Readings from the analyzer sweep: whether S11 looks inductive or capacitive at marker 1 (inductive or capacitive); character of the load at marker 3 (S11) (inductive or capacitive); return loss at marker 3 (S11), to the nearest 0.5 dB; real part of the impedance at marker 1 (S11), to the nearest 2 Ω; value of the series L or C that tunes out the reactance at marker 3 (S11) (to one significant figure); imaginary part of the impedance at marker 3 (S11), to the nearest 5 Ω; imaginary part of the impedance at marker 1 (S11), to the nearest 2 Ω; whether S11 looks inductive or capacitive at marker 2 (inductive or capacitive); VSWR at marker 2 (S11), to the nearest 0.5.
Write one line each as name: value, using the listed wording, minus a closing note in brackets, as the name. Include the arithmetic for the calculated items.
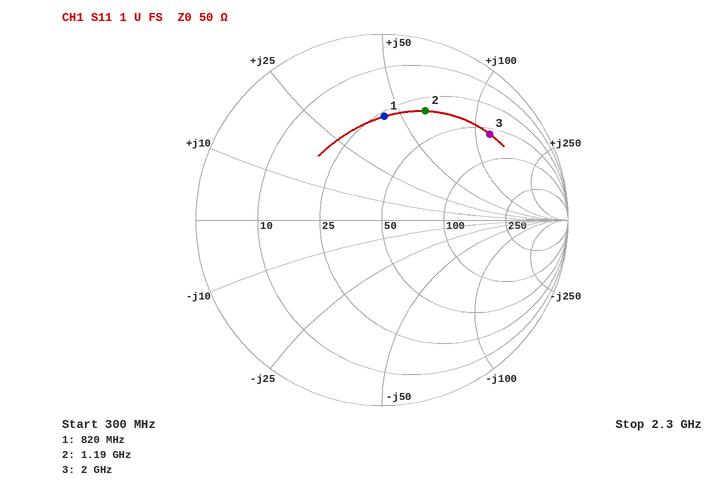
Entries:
whether S11 looks inductive or capacitive at marker 1: inductive
character of the load at marker 3 (S11): inductive
return loss at marker 3 (S11), to the nearest 0.5 dB: 2.5 dB
real part of the impedance at marker 1 (S11), to the nearest 2 Ω: 26 Ω
value of the series L or C that tunes out the reactance at marker 3 (S11): C = 1/(2π × 2 GHz × 120 Ω) ≈ 663 fF, so 700 fF to one significant figure
imaginary part of the impedance at marker 3 (S11), to the nearest 5 Ω: +120 Ω
imaginary part of the impedance at marker 1 (S11), to the nearest 2 Ω: +44 Ω
whether S11 looks inductive or capacitive at marker 2: inductive
VSWR at marker 2 (S11), to the nearest 0.5: 4.5
